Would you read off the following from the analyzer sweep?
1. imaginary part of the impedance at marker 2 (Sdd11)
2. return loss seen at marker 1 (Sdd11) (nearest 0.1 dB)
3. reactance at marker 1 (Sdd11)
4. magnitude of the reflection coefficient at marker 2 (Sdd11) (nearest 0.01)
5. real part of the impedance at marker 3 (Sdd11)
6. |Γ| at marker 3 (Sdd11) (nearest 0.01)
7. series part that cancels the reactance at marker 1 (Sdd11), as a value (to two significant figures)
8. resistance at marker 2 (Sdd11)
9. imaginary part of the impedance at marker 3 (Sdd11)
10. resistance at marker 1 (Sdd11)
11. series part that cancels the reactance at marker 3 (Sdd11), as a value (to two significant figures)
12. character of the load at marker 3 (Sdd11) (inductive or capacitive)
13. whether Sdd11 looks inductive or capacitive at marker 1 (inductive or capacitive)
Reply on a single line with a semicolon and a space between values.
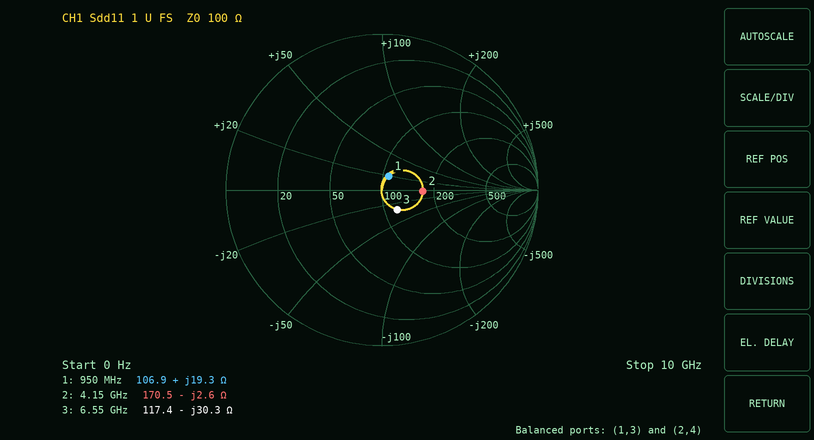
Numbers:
-2.6 Ω; 20.1 dB; +19.3 Ω; 0.26; 117.4 Ω; 0.16; 8.7 pF; 170.5 Ω; -30.3 Ω; 106.9 Ω; 740 pH; capacitive; inductive
